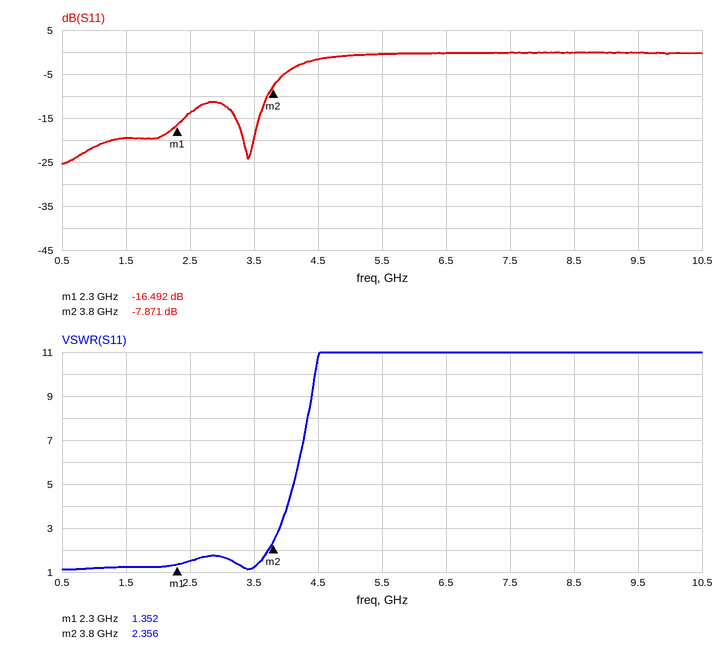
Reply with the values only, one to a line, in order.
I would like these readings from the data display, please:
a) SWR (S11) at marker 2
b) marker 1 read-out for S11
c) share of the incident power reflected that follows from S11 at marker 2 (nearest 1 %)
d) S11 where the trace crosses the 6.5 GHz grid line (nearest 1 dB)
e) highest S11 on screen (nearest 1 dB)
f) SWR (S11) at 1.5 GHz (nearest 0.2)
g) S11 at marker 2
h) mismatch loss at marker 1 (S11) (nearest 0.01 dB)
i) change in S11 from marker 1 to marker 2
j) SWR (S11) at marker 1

2.356
-16.492 dB
16 %
0 dB
0 dB
1.2
-7.871 dB
0.10 dB
8.621 dB
1.352
